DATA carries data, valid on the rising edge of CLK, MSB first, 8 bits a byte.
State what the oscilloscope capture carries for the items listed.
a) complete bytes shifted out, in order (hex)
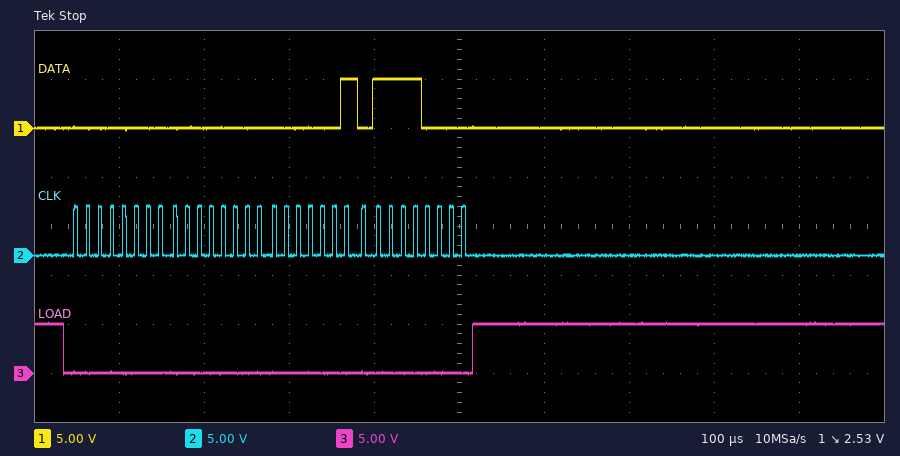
00 00 02 F0
